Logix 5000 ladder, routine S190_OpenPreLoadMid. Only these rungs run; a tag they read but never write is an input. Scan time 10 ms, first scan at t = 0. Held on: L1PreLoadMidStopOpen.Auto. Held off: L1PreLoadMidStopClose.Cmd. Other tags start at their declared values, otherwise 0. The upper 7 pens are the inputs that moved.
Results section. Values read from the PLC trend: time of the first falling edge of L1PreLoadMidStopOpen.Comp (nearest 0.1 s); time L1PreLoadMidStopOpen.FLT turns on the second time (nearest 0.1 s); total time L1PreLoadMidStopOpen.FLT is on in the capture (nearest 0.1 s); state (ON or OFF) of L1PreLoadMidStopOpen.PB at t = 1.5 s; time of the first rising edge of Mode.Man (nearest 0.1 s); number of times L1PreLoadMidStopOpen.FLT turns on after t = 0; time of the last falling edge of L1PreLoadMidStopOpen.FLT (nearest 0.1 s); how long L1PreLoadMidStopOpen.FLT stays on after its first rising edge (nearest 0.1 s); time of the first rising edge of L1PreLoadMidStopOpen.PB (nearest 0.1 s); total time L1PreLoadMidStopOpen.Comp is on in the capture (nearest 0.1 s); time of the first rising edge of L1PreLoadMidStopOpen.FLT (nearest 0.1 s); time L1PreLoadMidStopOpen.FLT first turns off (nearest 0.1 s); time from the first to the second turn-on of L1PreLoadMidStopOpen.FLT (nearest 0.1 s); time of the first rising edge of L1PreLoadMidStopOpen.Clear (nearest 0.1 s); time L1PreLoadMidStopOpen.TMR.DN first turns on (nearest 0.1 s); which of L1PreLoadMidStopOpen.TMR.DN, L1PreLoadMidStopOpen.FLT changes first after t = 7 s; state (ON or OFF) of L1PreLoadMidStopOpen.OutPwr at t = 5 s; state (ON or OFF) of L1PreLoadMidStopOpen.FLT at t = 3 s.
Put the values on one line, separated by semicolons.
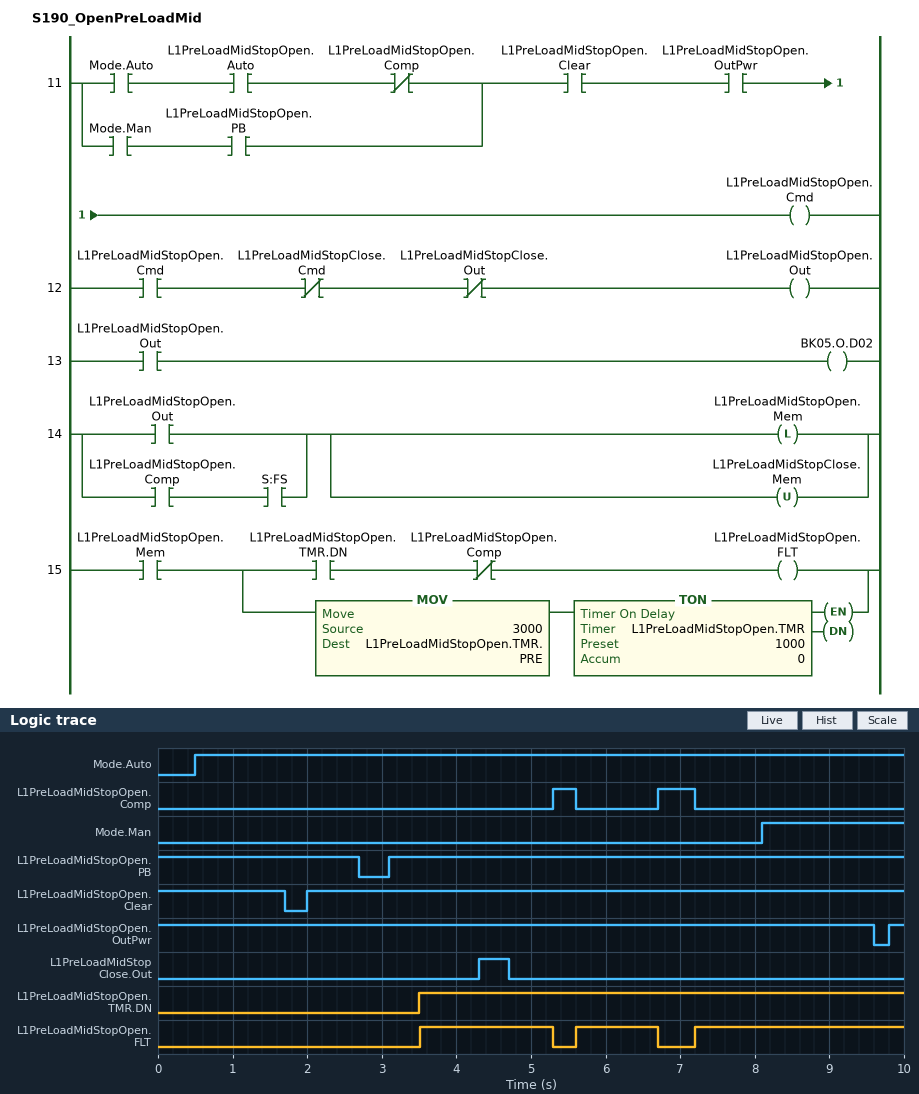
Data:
5.6 s; 5.6 s; 5.7 s; ON; 8.1 s; 3; 6.7 s; 1.8 s; 3.1 s; 0.8 s; 3.5 s; 5.3 s; 2.1 s; 2.0 s; 3.5 s; L1PreLoadMidStopOpen.FLT; ON; OFF
